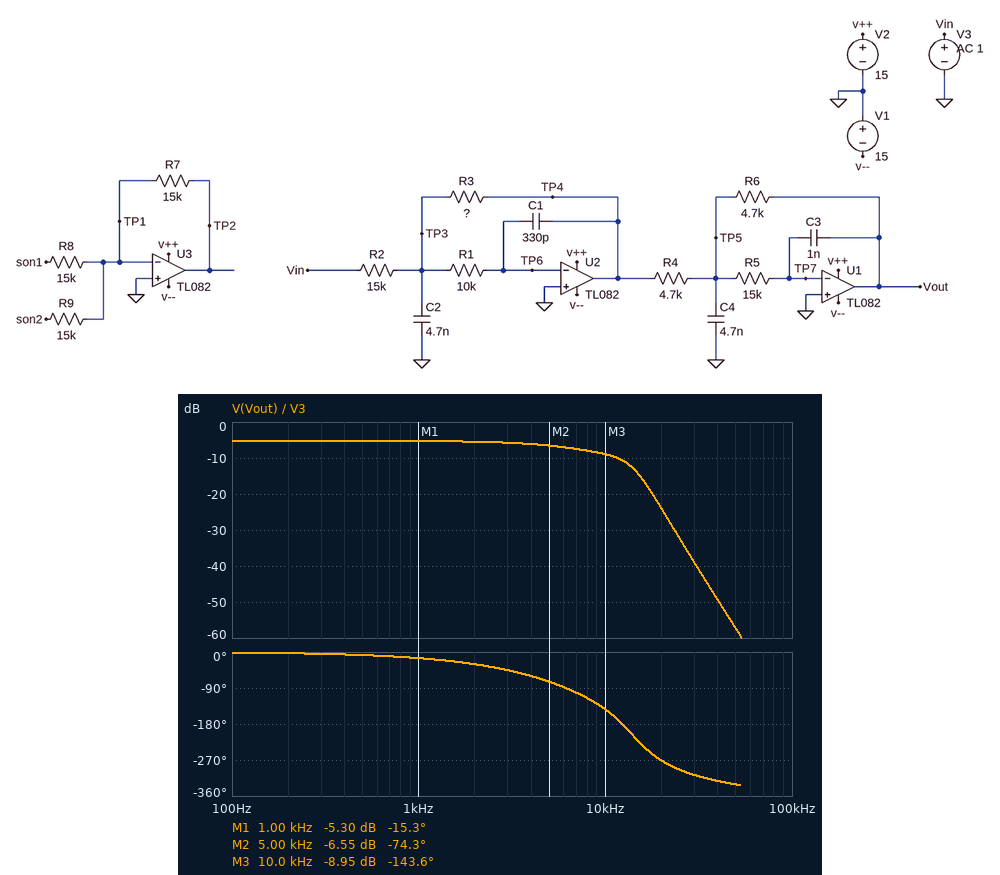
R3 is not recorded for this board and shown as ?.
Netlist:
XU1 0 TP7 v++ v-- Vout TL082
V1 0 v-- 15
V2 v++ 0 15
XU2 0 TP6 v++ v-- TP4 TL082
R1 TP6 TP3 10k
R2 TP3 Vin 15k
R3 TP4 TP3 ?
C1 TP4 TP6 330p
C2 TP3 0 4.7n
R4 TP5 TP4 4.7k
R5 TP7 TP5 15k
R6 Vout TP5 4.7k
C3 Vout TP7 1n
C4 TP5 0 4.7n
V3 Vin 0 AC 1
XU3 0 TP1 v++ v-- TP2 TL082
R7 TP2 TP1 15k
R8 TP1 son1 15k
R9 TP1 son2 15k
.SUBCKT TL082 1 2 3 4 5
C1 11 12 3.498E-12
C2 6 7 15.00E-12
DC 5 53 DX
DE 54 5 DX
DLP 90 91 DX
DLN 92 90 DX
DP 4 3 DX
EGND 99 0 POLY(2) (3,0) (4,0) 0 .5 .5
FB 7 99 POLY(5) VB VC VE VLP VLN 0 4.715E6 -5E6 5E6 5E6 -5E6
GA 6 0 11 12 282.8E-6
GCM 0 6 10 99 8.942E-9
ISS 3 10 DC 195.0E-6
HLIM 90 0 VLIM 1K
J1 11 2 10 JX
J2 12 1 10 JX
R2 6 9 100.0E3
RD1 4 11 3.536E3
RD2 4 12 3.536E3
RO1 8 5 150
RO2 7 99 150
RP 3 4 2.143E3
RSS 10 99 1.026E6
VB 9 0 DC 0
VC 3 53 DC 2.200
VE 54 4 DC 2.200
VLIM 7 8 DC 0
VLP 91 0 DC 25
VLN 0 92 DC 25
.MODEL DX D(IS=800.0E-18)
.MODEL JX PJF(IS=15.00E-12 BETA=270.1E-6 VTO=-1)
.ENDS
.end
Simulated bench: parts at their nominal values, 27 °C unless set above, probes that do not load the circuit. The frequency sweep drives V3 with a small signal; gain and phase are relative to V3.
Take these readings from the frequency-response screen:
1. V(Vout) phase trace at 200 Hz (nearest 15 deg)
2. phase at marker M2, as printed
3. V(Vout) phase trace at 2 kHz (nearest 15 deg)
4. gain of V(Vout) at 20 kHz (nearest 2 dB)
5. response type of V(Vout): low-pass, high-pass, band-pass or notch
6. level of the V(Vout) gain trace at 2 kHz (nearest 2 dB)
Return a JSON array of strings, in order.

["0 deg", "-74.3 deg", "-30 deg", "-24 dB", "low-pass", "-6 dB"]
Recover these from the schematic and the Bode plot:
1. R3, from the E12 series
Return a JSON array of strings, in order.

["8.2 kΩ"]
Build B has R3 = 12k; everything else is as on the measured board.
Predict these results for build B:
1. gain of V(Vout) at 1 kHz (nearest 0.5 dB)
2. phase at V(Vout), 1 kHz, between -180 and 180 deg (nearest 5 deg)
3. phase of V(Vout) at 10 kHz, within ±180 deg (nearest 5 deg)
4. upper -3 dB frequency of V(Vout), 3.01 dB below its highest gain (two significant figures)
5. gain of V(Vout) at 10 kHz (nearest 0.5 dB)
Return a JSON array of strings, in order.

["-2.0 dB", "-15 deg", "-165 deg", "9.5 kHz", "-5.5 dB"]
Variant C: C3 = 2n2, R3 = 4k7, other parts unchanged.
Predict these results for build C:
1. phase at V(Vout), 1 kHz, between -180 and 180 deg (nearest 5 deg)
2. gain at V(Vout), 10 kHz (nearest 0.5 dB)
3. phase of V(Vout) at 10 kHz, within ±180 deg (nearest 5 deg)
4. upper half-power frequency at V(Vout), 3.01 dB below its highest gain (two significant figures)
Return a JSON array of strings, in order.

["-30 deg", "-22.5 dB", "-140 deg", "2.4 kHz"]
